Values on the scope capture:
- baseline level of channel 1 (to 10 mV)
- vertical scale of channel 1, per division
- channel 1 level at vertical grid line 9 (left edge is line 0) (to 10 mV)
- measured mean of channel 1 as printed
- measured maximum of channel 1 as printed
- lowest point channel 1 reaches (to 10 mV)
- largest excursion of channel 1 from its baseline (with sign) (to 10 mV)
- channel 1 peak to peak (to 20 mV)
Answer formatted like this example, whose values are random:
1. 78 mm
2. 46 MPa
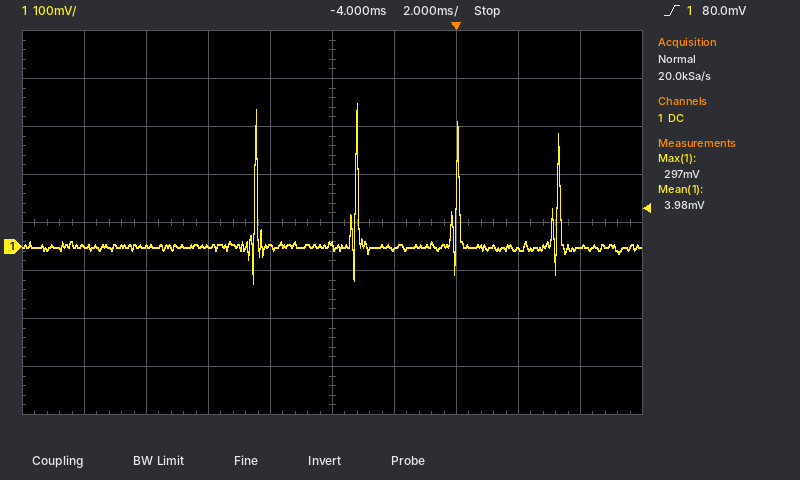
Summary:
1. 0 mV
2. 100 mV
3. 0 mV
4. 3.98 mV
5. 297 mV
6. -80 mV
7. +300 mV
8. 380 mV
